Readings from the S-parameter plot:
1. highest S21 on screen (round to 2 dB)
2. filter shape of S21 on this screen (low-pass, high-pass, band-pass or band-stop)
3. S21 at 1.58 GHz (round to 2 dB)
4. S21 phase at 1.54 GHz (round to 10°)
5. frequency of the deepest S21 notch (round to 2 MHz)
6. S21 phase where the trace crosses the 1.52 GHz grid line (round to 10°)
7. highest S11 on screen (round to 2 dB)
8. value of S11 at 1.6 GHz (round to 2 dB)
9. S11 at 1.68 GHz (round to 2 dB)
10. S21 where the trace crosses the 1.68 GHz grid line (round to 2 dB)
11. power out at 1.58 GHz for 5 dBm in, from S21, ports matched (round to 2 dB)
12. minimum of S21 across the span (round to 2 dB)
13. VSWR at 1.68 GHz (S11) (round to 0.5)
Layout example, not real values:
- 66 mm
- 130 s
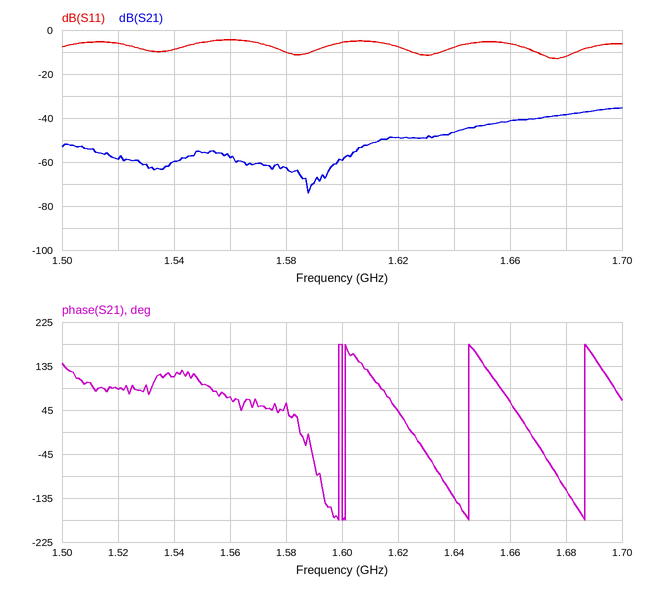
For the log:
- -36 dB
- high-pass
- -62 dB
- 110°
- 1.588 GHz
- 90°
- -4 dB
- -6 dB
- -12 dB
- -38 dB
- -58 dBm
- -74 dB
- 1.5
